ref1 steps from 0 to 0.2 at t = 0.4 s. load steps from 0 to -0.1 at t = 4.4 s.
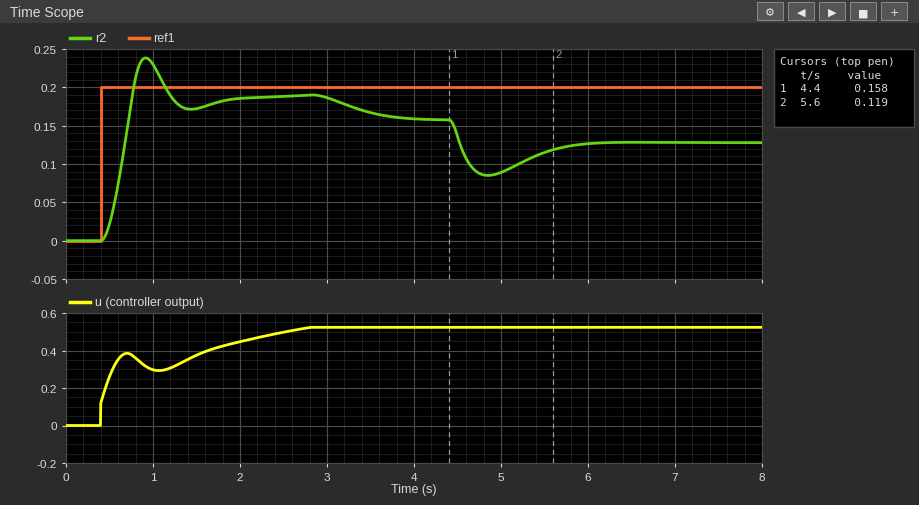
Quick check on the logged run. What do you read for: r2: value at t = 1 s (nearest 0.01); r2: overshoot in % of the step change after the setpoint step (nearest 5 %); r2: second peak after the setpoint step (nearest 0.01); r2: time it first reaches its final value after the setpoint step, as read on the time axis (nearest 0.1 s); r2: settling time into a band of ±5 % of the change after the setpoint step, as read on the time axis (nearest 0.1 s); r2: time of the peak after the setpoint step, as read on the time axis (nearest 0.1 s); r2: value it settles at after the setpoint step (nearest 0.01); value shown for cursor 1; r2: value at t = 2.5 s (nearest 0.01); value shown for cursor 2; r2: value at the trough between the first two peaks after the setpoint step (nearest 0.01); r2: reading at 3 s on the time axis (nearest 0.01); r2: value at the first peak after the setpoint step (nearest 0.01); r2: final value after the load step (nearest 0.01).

0.23
50 %
0.19
0.7 s
3.5 s
0.9 s
0.16
0.158
0.19
0.119
0.17
0.19
0.24
0.13
